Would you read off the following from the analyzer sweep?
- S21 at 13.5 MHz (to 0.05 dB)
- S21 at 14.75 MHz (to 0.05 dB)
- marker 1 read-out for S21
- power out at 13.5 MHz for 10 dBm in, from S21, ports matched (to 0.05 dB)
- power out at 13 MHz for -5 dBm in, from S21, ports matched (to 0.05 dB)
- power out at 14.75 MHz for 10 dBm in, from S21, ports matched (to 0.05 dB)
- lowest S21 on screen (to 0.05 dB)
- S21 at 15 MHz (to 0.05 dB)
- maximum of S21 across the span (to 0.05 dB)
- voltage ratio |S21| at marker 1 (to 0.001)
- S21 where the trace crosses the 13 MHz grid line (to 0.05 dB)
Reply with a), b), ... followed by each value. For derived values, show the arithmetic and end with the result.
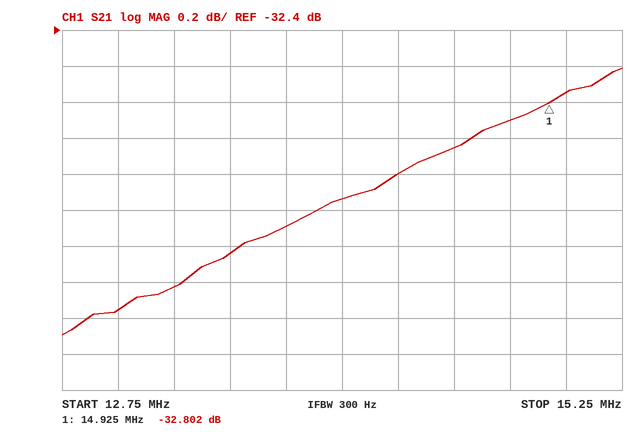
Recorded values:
a) -33.65 dB
b) -32.90 dB
c) -32.802 dB
d) 10 dBm + (-33.65 dB) = -23.65 dBm
e) -5 dBm + (-33.95 dB) = -38.95 dBm
f) 10 dBm + (-32.90 dB) = -22.90 dBm
g) -34.10 dB
h) -32.75 dB
i) -32.60 dB
j) 10^(-32.802/20) ≈ 0.023
k) -33.95 dB
